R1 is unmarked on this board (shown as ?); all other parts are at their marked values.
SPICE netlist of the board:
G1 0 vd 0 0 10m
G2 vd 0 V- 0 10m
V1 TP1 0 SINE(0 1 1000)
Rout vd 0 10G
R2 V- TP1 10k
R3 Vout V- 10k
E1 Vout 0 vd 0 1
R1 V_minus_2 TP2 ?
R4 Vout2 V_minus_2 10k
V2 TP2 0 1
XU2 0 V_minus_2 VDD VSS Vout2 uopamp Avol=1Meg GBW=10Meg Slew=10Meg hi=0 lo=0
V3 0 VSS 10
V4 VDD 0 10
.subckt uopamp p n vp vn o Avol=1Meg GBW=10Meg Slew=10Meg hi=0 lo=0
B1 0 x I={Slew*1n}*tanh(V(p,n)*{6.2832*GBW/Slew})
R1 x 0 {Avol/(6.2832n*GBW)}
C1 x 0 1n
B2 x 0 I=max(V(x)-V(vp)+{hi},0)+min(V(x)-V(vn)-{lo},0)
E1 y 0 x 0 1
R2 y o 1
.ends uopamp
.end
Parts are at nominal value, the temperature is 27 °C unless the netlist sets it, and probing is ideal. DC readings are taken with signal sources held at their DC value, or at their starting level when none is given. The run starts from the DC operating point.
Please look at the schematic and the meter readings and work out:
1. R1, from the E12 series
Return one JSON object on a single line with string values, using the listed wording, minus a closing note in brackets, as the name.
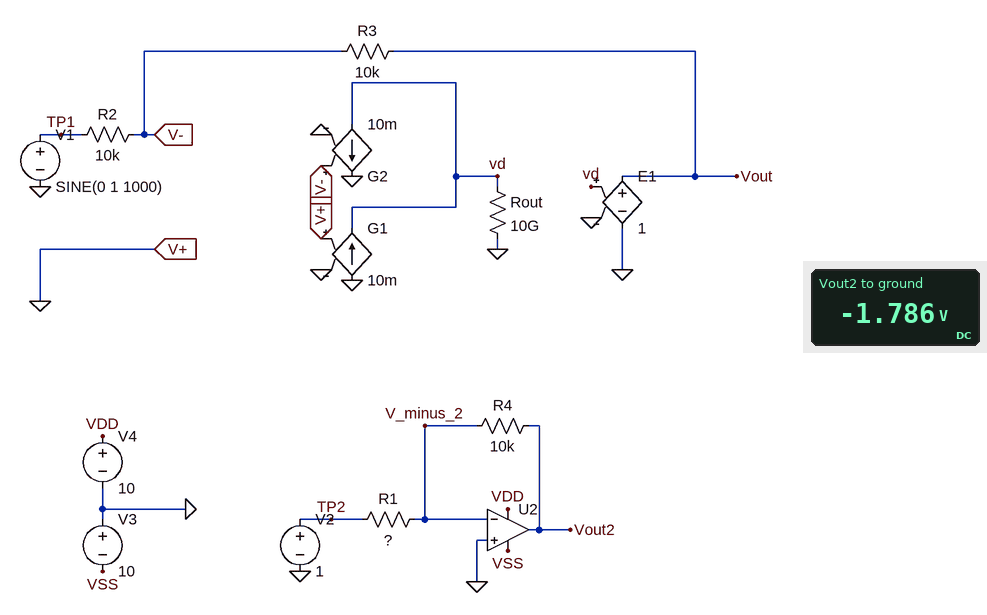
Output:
{"R1, from the E12 series": "5.6 kΩ"}
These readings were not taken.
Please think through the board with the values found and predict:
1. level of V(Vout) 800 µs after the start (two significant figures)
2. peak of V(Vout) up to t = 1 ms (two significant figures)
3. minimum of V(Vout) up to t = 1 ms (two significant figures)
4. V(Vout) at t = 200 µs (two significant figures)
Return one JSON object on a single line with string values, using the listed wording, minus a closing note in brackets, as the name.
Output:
{"level of V(Vout) 800 µs after the start": "950 mV", "peak of V(Vout) up to t = 1 ms": "1.0 V", "minimum of V(Vout) up to t = 1 ms": "-1.0 V", "V(Vout) at t = 200 µs": "-950 mV"}
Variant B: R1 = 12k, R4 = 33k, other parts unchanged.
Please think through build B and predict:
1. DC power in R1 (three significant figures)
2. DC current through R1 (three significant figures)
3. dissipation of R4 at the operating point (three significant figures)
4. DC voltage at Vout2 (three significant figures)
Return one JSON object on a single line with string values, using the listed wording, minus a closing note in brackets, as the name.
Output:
{"DC power in R1": "83.3 µW", "DC current through R1": "83.3 µA", "dissipation of R4 at the operating point": "229 µW", "DC voltage at Vout2": "-2.75 V"}
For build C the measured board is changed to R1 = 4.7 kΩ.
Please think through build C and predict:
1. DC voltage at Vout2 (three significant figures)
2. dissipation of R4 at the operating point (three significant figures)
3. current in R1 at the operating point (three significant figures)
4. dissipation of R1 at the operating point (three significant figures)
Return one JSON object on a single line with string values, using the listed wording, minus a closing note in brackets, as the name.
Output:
{"DC voltage at Vout2": "-2.13 V", "dissipation of R4 at the operating point": "453 µW", "current in R1 at the operating point": "213 µA", "dissipation of R1 at the operating point": "213 µW"}
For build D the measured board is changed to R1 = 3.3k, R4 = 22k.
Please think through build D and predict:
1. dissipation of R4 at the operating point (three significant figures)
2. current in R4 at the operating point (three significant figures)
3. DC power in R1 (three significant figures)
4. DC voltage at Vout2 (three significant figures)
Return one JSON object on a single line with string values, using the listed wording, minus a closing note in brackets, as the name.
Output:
{"dissipation of R4 at the operating point": "2.02 mW", "current in R4 at the operating point": "303 µA", "DC power in R1": "303 µW", "DC voltage at Vout2": "-6.67 V"}
